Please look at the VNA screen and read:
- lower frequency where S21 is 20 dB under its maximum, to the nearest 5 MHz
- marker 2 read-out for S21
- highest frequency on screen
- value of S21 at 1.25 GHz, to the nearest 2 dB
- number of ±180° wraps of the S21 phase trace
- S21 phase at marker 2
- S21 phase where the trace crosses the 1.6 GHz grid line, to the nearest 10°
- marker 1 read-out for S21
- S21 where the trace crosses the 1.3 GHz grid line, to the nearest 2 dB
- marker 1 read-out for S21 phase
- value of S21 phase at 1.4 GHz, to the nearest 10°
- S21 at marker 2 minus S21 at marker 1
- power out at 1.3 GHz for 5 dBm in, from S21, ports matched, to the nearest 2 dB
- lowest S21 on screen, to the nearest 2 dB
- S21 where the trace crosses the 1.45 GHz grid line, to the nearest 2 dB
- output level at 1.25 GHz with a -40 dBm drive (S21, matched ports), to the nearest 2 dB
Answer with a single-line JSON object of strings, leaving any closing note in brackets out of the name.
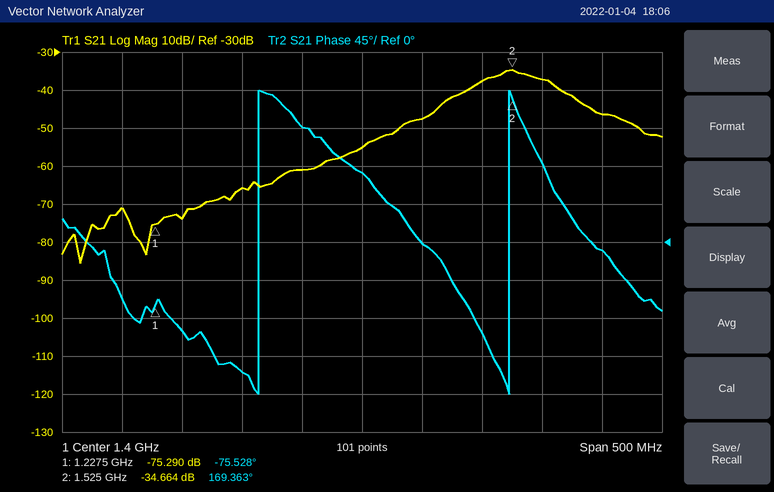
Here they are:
{"lower frequency where S21 is 20 dB under its maximum, to the nearest 5 MHz": "1.400 GHz", "marker 2 read-out for S21": "-34.664 dB", "highest frequency on screen": "1.65 GHz", "value of S21 at 1.25 GHz, to the nearest 2 dB": "-74 dB", "number of ±180° wraps of the S21 phase trace": "2", "S21 phase at marker 2": "169.363°", "S21 phase where the trace crosses the 1.6 GHz grid line, to the nearest 10°": "-10°", "marker 1 read-out for S21": "-75.290 dB", "S21 where the trace crosses the 1.3 GHz grid line, to the nearest 2 dB": "-66 dB", "marker 1 read-out for S21 phase": "-75.528°", "value of S21 phase at 1.4 GHz, to the nearest 10°": "80°", "S21 at marker 2 minus S21 at marker 1": "40.626 dB", "power out at 1.3 GHz for 5 dBm in, from S21, ports matched, to the nearest 2 dB": "-60 dBm", "lowest S21 on screen, to the nearest 2 dB": "-86 dB", "S21 where the trace crosses the 1.45 GHz grid line, to the nearest 2 dB": "-48 dB", "output level at 1.25 GHz with a -40 dBm drive (S21, matched ports), to the nearest 2 dB": "-114 dBm"}
